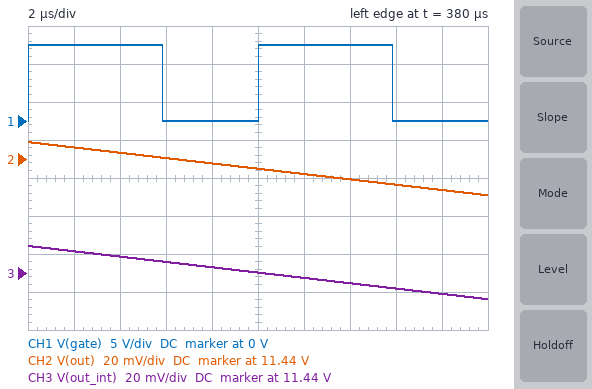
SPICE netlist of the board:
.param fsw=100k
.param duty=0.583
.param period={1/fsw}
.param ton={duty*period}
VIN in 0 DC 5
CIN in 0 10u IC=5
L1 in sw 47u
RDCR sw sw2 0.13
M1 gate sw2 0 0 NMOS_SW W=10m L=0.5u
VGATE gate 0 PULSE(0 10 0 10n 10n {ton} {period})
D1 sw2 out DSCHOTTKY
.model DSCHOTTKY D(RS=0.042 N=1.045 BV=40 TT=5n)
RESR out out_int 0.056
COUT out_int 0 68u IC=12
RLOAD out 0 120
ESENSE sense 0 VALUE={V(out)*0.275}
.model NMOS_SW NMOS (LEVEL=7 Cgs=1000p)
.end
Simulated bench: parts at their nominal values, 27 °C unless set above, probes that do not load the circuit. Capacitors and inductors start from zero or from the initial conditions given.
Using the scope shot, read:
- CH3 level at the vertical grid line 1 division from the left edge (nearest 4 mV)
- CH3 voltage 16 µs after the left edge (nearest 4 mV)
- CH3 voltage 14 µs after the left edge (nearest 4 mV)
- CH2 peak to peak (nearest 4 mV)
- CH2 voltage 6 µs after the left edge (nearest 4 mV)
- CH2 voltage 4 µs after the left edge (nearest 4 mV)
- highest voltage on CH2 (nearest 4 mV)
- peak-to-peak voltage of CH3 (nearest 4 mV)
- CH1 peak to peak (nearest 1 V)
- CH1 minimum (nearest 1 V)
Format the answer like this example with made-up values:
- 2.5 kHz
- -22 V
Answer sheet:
- 11.452 V
- 11.432 V
- 11.436 V
- 28 mV
- 11.440 V
- 11.444 V
- 11.448 V
- 28 mV
- 10 V
- 0 V
